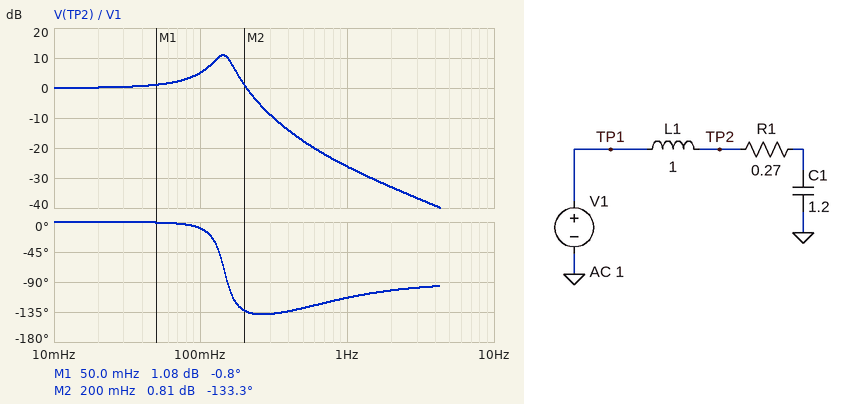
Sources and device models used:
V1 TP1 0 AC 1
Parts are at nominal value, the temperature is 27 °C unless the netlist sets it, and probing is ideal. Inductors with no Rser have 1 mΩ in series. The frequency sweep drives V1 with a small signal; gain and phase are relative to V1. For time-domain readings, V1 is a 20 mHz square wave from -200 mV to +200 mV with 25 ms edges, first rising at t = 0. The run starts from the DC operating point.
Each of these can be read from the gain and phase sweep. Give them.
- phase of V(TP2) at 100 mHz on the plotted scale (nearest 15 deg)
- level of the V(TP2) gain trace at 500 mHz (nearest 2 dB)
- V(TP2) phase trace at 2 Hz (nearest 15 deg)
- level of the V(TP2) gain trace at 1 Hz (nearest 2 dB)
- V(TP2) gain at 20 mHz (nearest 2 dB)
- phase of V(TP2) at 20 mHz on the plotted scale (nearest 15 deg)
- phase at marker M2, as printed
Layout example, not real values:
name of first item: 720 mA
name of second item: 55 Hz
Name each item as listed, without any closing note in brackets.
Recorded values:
phase of V(TP2) at 100 mHz on the plotted scale: -15 deg
level of the V(TP2) gain trace at 500 mHz: -18 dB
V(TP2) phase trace at 2 Hz: -105 deg
level of the V(TP2) gain trace at 1 Hz: -26 dB
V(TP2) gain at 20 mHz: 0 dB
phase of V(TP2) at 20 mHz on the plotted scale: 0 deg
phase at marker M2, as printed: -133.3 deg
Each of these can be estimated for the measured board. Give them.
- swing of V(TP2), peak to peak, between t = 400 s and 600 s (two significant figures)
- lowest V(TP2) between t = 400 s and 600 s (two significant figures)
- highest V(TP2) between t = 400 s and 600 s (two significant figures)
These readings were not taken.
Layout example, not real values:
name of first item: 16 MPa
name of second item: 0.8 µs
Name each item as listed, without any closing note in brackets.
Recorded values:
swing of V(TP2), peak to peak, between t = 400 s and 600 s: 940 mV
lowest V(TP2) between t = 400 s and 600 s: -470 mV
highest V(TP2) between t = 400 s and 600 s: 470 mV
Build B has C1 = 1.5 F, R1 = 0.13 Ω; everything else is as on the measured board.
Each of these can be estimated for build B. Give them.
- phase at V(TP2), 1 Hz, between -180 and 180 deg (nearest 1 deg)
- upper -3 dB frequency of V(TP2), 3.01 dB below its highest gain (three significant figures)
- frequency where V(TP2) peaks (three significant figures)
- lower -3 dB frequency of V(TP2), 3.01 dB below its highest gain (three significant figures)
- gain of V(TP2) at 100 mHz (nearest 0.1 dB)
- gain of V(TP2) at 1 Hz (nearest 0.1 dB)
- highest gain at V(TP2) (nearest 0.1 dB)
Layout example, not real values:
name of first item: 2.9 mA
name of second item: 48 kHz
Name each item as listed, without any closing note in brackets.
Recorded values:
phase at V(TP2), 1 Hz, between -180 and 180 deg: -128 deg
upper -3 dB frequency of V(TP2), 3.01 dB below its highest gain: 139 mHz
frequency where V(TP2) peaks: 129 mHz
lower -3 dB frequency of V(TP2), 3.01 dB below its highest gain: 118 mHz
gain of V(TP2) at 100 mHz: 7.5 dB
gain of V(TP2) at 1 Hz: -31.3 dB
highest gain at V(TP2): 16.0 dB
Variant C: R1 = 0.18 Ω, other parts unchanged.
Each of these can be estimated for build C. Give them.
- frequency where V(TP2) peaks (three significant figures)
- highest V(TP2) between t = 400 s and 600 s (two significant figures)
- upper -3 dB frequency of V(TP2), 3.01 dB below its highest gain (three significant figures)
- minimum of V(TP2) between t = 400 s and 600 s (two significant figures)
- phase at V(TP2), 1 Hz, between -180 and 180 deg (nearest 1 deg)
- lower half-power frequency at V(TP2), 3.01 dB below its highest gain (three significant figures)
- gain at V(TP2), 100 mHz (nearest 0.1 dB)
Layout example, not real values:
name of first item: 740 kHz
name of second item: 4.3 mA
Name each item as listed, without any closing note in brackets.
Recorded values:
frequency where V(TP2) peaks: 144 mHz
highest V(TP2) between t = 400 s and 600 s: 530 mV
upper -3 dB frequency of V(TP2), 3.01 dB below its highest gain: 158 mHz
minimum of V(TP2) between t = 400 s and 600 s: -530 mV
phase at V(TP2), 1 Hz, between -180 and 180 deg: -125 deg
lower half-power frequency at V(TP2), 3.01 dB below its highest gain: 129 mHz
gain at V(TP2), 100 mHz: 5.4 dB
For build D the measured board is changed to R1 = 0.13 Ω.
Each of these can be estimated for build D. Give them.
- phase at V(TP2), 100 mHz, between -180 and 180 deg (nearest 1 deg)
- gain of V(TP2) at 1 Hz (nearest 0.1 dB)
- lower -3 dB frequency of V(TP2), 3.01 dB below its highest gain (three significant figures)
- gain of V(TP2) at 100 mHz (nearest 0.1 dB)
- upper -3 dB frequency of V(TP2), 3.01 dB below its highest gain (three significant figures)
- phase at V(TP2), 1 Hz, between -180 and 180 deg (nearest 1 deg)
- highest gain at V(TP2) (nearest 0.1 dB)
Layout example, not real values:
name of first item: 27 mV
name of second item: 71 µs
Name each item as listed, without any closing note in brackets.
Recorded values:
phase at V(TP2), 100 mHz, between -180 and 180 deg: -5 deg
gain of V(TP2) at 1 Hz: -30.4 dB
lower -3 dB frequency of V(TP2), 3.01 dB below its highest gain: 134 mHz
gain of V(TP2) at 100 mHz: 5.5 dB
upper -3 dB frequency of V(TP2), 3.01 dB below its highest gain: 155 mHz
phase at V(TP2), 1 Hz, between -180 and 180 deg: -134 deg
highest gain at V(TP2): 17.0 dB
